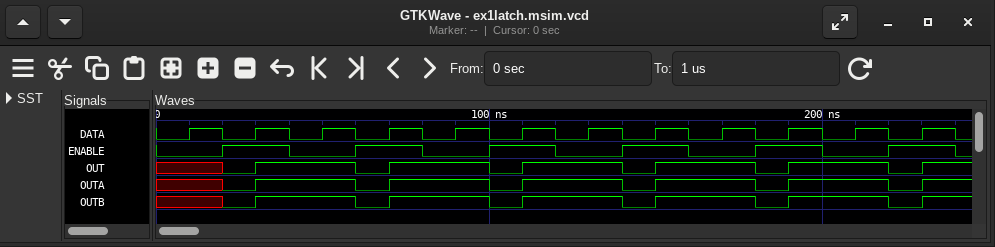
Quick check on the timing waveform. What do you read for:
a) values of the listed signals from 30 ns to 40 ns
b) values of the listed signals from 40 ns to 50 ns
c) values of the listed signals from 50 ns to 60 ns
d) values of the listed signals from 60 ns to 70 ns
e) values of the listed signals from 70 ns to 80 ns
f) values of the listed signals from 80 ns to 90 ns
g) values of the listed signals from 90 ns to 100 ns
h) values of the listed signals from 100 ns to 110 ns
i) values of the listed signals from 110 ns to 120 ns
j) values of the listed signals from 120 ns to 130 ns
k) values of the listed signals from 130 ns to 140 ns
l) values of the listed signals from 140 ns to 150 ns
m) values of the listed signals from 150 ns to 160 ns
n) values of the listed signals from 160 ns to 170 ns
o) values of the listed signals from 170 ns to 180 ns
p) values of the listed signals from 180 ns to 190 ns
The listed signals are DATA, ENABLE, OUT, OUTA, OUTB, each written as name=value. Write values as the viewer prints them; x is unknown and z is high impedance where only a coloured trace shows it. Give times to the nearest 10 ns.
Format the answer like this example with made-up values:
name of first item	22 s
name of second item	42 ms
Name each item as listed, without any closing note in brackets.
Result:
values of the listed signals from 30 ns to 40 ns	DATA=1, ENABLE=1, OUT=1, OUTA=1, OUTB=1
values of the listed signals from 40 ns to 50 ns	DATA=0, ENABLE=0, OUT=1, OUTA=1, OUTB=1
values of the listed signals from 50 ns to 60 ns	DATA=1, ENABLE=0, OUT=1, OUTA=1, OUTB=1
values of the listed signals from 60 ns to 70 ns	DATA=0, ENABLE=1, OUT=0, OUTA=0, OUTB=0
values of the listed signals from 70 ns to 80 ns	DATA=1, ENABLE=1, OUT=1, OUTA=1, OUTB=1
values of the listed signals from 80 ns to 90 ns	DATA=0, ENABLE=0, OUT=1, OUTA=1, OUTB=1
values of the listed signals from 90 ns to 100 ns	DATA=1, ENABLE=0, OUT=1, OUTA=1, OUTB=1
values of the listed signals from 100 ns to 110 ns	DATA=0, ENABLE=1, OUT=0, OUTA=0, OUTB=0
values of the listed signals from 110 ns to 120 ns	DATA=1, ENABLE=1, OUT=1, OUTA=1, OUTB=1
values of the listed signals from 120 ns to 130 ns	DATA=0, ENABLE=0, OUT=1, OUTA=1, OUTB=1
values of the listed signals from 130 ns to 140 ns	DATA=1, ENABLE=0, OUT=1, OUTA=1, OUTB=1
values of the listed signals from 140 ns to 150 ns	DATA=0, ENABLE=1, OUT=0, OUTA=0, OUTB=0
values of the listed signals from 150 ns to 160 ns	DATA=1, ENABLE=1, OUT=1, OUTA=1, OUTB=1
values of the listed signals from 160 ns to 170 ns	DATA=0, ENABLE=0, OUT=1, OUTA=1, OUTB=1
values of the listed signals from 170 ns to 180 ns	DATA=1, ENABLE=0, OUT=1, OUTA=1, OUTB=1
values of the listed signals from 180 ns to 190 ns	DATA=0, ENABLE=1, OUT=0, OUTA=0, OUTB=0
